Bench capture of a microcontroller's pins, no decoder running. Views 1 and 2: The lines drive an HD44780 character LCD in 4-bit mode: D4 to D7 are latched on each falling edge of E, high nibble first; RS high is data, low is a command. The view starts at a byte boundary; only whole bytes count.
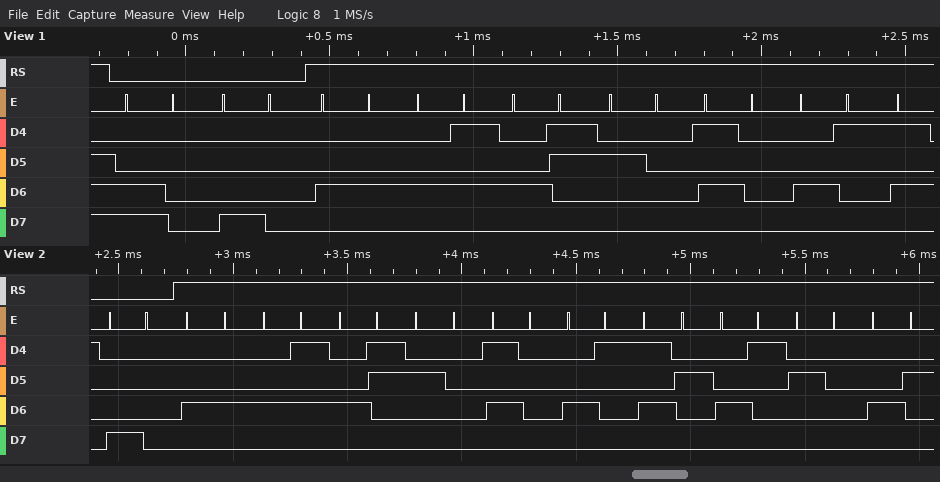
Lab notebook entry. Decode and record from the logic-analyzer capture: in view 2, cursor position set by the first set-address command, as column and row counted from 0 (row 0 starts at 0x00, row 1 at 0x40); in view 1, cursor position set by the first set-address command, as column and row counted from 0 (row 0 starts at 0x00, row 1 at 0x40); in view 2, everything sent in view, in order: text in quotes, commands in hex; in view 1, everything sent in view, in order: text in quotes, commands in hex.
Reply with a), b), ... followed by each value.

a) column 0, row 0
b) column 0, row 1
c) 0x80 "DEC PARA B"
d) 0xC0 0x80 "DEC PA"
